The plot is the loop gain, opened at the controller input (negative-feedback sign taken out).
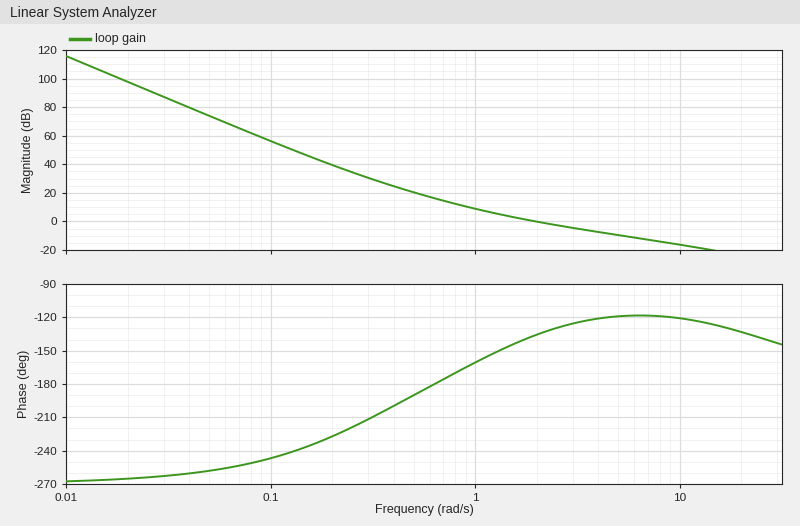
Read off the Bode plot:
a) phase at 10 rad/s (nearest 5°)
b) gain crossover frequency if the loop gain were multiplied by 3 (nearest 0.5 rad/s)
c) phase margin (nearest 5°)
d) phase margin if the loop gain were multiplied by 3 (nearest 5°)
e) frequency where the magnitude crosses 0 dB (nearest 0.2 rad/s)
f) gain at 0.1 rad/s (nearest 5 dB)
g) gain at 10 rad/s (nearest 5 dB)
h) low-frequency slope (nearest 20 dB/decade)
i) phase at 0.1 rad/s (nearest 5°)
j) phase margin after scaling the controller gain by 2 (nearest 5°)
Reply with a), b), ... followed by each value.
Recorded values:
a) -120°
b) 5.0 rad/s
c) 45°
d) 60°
e) 2.0 rad/s
f) 55 dB
g) -15 dB
h) -60 dB/decade
i) -245°
j) 55°
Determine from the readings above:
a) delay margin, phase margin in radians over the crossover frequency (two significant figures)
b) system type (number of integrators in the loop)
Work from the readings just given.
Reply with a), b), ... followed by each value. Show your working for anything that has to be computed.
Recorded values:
a) 45 × π / 180 / 2 = 0.39 s
b) 3
